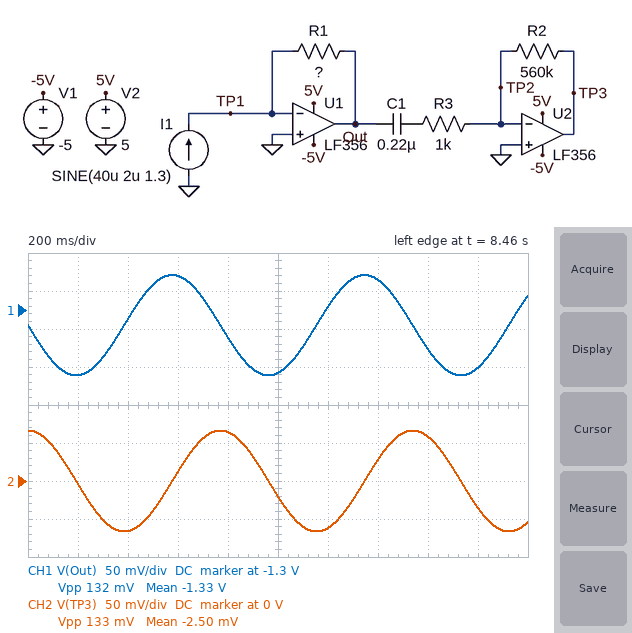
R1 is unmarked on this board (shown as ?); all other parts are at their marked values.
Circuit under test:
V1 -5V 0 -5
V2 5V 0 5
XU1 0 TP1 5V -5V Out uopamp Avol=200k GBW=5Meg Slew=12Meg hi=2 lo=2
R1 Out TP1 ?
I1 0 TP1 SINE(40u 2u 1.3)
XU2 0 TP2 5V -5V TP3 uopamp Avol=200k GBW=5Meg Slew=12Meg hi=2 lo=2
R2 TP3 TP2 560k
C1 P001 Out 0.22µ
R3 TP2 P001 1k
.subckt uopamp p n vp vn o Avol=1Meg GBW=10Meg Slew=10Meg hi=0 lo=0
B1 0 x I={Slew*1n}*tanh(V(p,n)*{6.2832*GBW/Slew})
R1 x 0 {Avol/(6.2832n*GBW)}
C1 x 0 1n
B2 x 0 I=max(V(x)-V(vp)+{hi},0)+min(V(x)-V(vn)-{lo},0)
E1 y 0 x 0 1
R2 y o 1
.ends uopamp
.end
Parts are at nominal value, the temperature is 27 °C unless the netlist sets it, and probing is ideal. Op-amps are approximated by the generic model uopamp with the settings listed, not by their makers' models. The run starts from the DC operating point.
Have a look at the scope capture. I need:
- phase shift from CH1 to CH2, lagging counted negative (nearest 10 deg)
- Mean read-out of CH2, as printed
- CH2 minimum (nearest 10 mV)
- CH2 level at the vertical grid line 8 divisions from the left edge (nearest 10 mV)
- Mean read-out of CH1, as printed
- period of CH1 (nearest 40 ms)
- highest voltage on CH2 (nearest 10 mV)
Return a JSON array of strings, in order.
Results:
["-90 deg", "-2.50 mV", "-70 mV", "60 mV", "-1.33 V", "760 ms", "70 mV"]
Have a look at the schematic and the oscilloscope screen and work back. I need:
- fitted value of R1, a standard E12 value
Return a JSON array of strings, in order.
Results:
["33 kΩ"]
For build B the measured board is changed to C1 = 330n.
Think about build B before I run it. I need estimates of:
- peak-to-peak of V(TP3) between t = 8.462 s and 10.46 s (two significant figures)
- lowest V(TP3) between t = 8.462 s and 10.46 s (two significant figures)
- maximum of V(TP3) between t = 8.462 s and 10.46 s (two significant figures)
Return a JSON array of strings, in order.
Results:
["200 mV", "-100 mV", "100 mV"]
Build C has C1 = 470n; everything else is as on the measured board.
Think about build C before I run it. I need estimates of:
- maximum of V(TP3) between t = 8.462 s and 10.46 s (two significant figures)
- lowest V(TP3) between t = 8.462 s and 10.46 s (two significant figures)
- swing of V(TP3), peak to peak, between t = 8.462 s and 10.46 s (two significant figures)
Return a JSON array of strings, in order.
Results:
["140 mV", "-140 mV", "280 mV"]
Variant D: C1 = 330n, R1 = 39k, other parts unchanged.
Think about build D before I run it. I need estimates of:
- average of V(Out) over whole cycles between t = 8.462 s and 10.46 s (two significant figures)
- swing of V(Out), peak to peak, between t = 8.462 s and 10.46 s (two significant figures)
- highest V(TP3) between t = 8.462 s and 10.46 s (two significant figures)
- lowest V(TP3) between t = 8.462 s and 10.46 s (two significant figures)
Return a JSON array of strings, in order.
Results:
["-1.6 V", "160 mV", "120 mV", "-120 mV"]
